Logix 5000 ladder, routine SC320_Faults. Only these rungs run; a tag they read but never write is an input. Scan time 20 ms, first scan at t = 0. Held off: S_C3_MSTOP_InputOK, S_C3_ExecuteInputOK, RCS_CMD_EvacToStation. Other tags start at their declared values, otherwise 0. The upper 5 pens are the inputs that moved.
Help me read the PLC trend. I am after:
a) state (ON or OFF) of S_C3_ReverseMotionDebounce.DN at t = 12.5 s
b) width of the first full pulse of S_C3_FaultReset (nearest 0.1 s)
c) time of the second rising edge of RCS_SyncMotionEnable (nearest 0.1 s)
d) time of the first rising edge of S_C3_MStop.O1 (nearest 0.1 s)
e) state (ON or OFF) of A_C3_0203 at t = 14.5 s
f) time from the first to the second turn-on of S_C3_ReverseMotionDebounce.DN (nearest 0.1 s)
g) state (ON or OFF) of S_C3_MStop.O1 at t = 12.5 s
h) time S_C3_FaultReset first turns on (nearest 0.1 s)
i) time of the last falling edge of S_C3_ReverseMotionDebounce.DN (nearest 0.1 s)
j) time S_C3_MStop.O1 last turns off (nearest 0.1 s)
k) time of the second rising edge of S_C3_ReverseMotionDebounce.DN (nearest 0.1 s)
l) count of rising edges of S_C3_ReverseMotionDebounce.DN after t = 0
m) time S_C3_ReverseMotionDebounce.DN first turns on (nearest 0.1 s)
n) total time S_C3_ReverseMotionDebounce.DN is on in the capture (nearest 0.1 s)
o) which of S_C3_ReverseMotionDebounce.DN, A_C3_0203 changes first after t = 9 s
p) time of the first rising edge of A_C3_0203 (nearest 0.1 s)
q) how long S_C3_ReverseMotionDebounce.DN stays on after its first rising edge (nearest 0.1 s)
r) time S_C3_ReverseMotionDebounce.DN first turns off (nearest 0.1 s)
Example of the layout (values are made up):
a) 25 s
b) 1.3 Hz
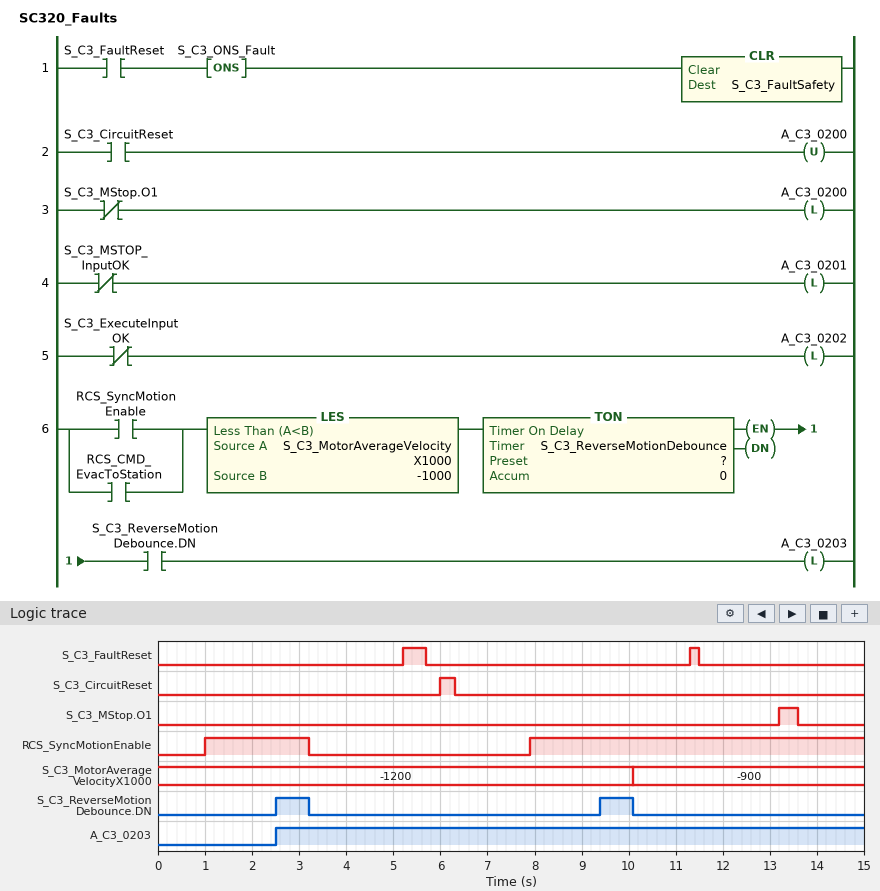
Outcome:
a) OFF
b) 0.5 s
c) 7.9 s
d) 13.2 s
e) ON
f) 6.9 s
g) OFF
h) 5.2 s
i) 10.1 s
j) 13.6 s
k) 9.4 s
l) 2
m) 2.5 s
n) 1.4 s
o) S_C3_ReverseMotionDebounce.DN
p) 2.5 s
q) 0.7 s
r) 3.2 s
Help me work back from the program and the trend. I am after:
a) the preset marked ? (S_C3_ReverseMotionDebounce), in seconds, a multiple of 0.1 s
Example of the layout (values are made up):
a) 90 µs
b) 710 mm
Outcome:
a) 1.5 s
